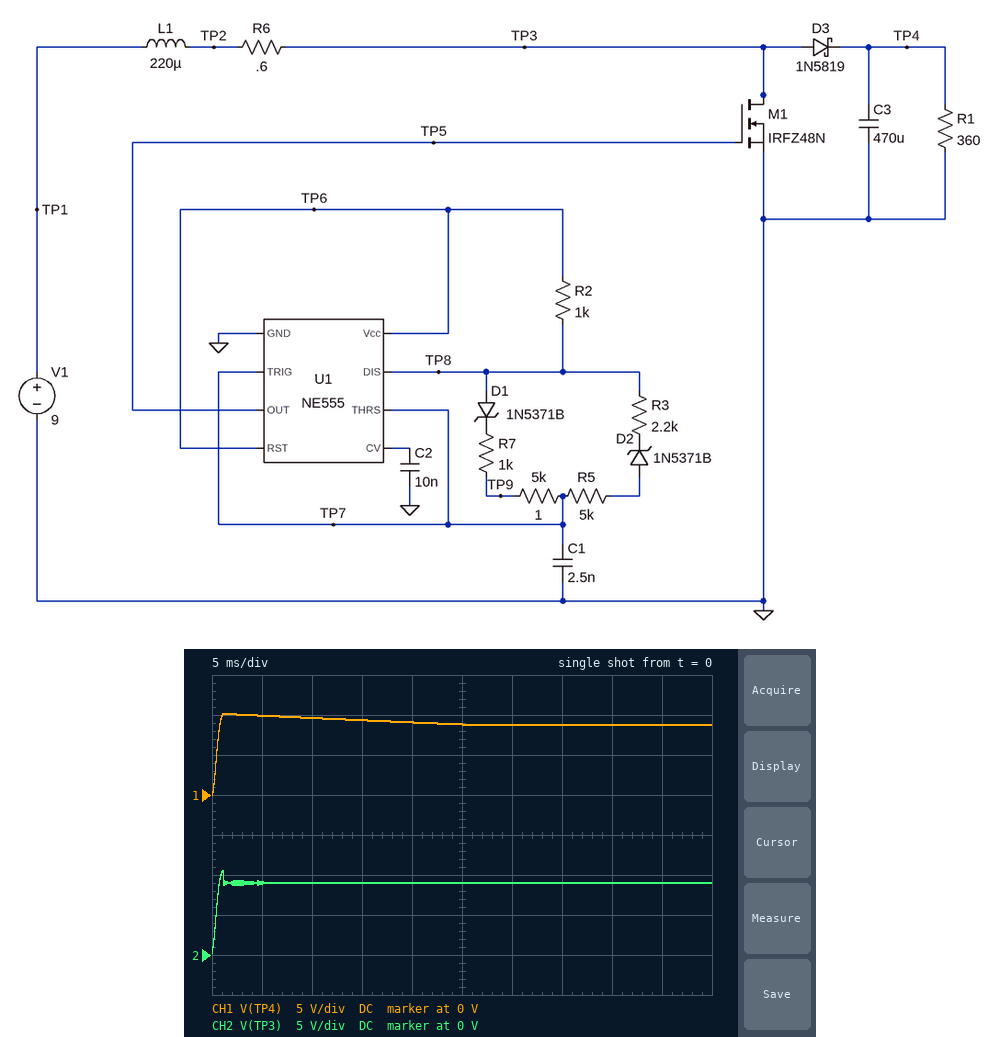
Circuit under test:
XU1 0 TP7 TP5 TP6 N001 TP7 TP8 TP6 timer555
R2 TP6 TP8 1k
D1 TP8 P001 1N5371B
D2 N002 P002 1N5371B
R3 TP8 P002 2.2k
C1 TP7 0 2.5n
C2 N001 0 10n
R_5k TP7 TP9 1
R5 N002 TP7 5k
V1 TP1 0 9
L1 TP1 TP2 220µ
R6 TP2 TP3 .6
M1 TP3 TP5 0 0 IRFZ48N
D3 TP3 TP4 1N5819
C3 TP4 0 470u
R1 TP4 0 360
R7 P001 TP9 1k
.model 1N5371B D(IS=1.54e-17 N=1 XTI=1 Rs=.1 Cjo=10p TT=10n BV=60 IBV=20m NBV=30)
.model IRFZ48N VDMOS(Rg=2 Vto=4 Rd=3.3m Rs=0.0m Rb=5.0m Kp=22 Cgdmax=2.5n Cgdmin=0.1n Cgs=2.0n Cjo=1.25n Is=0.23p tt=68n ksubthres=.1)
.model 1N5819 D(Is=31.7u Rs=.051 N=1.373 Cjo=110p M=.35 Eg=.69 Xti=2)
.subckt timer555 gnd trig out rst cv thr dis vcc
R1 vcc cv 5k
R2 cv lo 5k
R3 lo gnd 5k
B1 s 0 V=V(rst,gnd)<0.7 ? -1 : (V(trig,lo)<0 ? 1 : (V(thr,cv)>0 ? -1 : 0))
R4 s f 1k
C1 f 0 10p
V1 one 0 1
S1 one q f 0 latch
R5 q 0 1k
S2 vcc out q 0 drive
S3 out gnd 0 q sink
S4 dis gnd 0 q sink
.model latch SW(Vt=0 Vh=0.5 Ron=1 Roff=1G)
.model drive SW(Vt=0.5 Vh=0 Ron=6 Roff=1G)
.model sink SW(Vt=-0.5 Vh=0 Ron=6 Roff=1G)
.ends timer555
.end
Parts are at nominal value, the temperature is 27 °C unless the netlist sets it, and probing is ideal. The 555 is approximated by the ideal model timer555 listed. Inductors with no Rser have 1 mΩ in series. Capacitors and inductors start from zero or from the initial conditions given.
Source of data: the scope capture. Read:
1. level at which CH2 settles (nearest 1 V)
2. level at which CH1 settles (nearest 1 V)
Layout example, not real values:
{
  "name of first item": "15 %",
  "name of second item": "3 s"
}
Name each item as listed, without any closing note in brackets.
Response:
{
  "level at which CH2 settles": "9 V",
  "level at which CH1 settles": "9 V"
}
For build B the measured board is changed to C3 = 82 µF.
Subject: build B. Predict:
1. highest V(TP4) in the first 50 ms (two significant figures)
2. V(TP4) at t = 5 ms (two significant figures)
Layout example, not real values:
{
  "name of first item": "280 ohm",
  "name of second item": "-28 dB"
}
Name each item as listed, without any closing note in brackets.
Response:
{
  "highest V(TP4) in the first 50 ms": "13 V",
  "V(TP4) at t = 5 ms": "11 V"
}
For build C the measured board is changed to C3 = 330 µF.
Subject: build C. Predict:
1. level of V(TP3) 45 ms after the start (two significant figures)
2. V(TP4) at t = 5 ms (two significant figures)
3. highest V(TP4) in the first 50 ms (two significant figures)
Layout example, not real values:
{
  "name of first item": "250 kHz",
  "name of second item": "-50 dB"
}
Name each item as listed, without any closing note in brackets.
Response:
{
  "level of V(TP3) 45 ms after the start": "9.0 V",
  "V(TP4) at t = 5 ms": "10 V",
  "highest V(TP4) in the first 50 ms": "11 V"
}
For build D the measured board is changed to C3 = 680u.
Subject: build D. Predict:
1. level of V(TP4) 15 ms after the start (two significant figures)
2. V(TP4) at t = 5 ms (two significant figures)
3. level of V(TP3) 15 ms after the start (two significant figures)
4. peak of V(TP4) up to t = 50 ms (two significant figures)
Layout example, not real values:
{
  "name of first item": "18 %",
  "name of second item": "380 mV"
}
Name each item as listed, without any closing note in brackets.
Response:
{
  "level of V(TP4) 15 ms after the start": "9.0 V",
  "V(TP4) at t = 5 ms": "9.4 V",
  "level of V(TP3) 15 ms after the start": "9.0 V",
  "peak of V(TP4) up to t = 50 ms": "9.5 V"
}
